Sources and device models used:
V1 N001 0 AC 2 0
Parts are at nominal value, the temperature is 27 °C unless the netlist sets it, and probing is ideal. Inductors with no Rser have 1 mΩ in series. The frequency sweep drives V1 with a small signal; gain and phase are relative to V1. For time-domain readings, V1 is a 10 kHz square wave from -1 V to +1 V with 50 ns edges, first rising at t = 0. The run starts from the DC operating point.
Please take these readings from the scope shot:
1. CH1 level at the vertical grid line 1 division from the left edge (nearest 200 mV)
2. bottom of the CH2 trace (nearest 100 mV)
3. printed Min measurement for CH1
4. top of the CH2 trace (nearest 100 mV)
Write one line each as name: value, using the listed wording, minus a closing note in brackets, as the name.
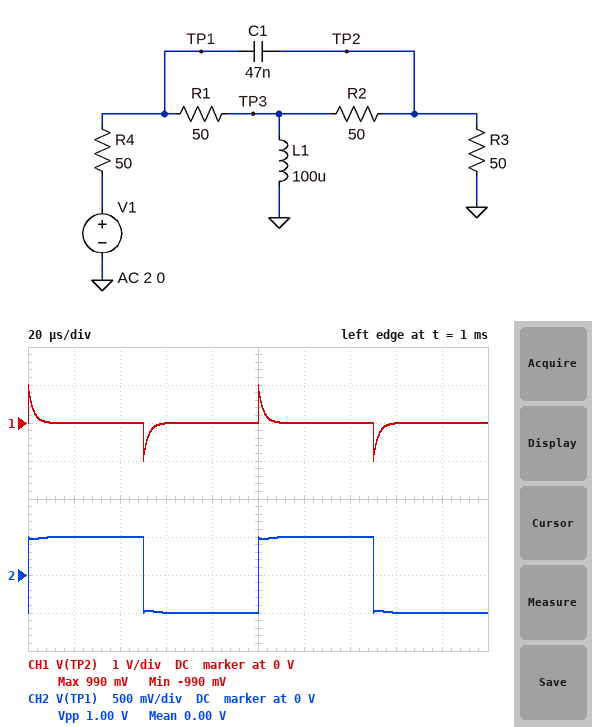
CH1 level at the vertical grid line 1 division from the left edge: 0 V
bottom of the CH2 trace: -500 mV
printed Min measurement for CH1: -990 mV
top of the CH2 trace: 500 mV
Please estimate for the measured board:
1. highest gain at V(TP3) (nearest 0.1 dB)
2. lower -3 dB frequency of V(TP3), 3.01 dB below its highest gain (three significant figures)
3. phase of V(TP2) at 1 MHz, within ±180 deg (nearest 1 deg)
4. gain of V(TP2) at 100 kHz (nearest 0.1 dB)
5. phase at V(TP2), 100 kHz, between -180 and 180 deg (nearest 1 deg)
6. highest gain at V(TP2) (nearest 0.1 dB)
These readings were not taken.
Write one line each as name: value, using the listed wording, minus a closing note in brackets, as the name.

highest gain at V(TP3): -6.0 dB
lower -3 dB frequency of V(TP3), 3.01 dB below its highest gain: 79.6 kHz
phase of V(TP2) at 1 MHz, within ±180 deg: 4 deg
gain of V(TP2) at 100 kHz: -7.9 dB
phase at V(TP2), 100 kHz, between -180 and 180 deg: 36 deg
highest gain at V(TP2): -6.0 dB
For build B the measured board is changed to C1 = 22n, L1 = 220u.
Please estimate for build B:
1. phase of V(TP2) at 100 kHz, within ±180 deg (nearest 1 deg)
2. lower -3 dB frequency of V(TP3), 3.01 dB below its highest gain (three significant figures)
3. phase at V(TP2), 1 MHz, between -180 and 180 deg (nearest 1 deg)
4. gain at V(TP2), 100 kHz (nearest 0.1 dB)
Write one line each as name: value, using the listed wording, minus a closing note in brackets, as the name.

phase of V(TP2) at 100 kHz, within ±180 deg: 33 deg
lower -3 dB frequency of V(TP3), 3.01 dB below its highest gain: 36.2 kHz
phase at V(TP2), 1 MHz, between -180 and 180 deg: 5 deg
gain at V(TP2), 100 kHz: -8.9 dB
